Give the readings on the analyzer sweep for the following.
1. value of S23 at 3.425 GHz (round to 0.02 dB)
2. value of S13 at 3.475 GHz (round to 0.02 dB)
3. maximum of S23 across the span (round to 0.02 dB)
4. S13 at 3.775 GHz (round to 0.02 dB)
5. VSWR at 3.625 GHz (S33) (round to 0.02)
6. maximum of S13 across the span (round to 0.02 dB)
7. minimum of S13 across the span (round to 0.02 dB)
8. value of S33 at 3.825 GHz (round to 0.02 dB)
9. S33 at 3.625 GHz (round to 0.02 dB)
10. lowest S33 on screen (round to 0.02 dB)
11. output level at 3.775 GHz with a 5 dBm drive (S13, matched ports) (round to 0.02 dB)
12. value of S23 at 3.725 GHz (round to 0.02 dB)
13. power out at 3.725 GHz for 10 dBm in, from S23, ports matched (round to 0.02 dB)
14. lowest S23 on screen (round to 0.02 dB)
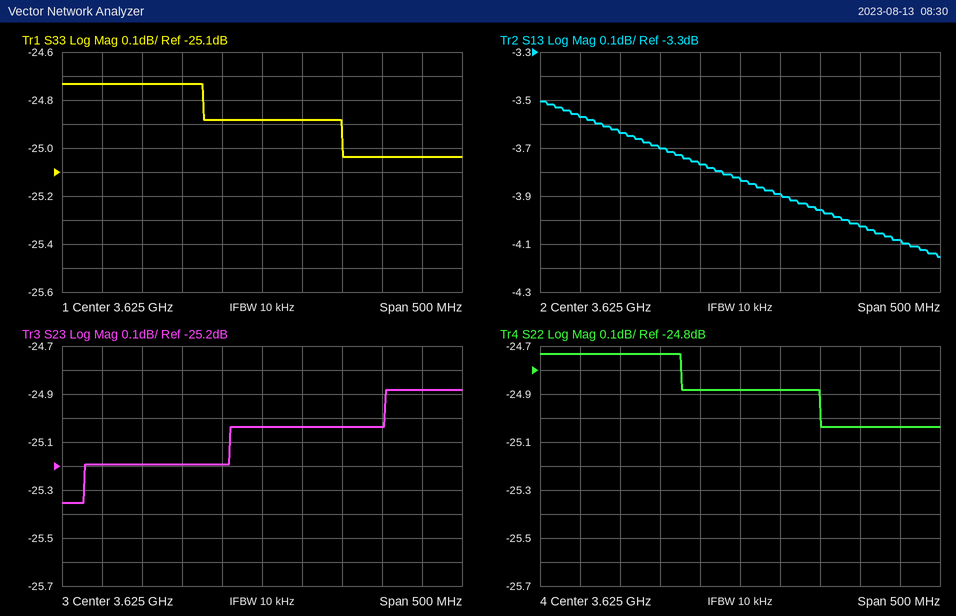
-25.20 dB
-3.64 dB
-24.88 dB
-4.02 dB
1.12
-3.50 dB
-4.16 dB
-25.04 dB
-24.88 dB
-25.04 dB
0.98 dBm
-25.04 dB
-15.04 dBm
-25.36 dB
